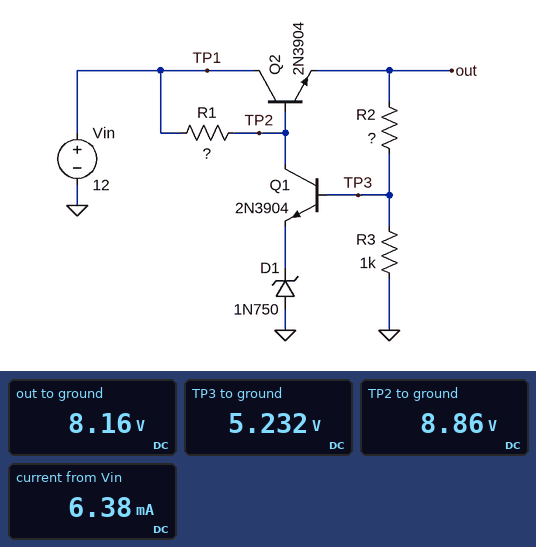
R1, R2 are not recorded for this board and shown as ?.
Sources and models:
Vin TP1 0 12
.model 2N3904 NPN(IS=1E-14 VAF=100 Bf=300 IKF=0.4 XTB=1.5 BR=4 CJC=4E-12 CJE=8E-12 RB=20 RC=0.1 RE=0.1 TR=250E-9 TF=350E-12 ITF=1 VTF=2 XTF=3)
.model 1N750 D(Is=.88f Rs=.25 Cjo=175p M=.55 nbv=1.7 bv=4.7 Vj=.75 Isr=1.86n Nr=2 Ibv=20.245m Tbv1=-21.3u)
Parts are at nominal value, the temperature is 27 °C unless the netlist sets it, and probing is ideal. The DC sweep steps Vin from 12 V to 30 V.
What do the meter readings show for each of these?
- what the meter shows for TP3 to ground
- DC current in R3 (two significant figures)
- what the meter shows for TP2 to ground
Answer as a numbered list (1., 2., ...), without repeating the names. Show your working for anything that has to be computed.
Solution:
1. 5.232 V
2. (5.232 V) / 1 kΩ = 5.2 mA
3. 8.86 V
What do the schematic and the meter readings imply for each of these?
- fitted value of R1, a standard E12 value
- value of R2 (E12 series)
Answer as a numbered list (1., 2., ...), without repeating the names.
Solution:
1. 2.7 kΩ
2. 560 Ω
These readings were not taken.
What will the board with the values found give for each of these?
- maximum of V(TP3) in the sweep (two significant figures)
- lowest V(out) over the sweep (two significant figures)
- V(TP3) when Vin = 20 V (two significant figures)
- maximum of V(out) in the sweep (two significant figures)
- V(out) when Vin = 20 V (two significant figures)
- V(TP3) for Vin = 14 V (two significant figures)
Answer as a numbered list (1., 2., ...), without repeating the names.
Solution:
1. 5.4 V
2. 8.2 V
3. 5.3 V
4. 8.4 V
5. 8.3 V
6. 5.3 V
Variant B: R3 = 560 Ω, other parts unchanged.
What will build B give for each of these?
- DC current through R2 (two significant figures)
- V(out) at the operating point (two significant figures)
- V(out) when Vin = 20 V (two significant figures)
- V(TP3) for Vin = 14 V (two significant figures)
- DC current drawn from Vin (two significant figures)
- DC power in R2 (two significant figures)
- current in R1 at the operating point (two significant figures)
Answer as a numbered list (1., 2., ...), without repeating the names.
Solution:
1. 9.2 mA
2. 10 V
3. 11 V
4. 5.2 V
5. 9.5 mA
6. 47 mW
7. 370 µA
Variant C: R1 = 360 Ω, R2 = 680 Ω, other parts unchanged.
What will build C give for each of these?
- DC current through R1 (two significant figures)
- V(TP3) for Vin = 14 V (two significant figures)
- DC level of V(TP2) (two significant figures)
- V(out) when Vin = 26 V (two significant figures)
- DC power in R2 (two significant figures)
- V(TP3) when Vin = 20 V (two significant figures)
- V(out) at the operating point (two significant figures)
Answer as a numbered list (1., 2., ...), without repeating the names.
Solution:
1. 6.4 mA
2. 5.4 V
3. 9.7 V
4. 9.4 V
5. 20 mW
6. 5.5 V
7. 9.0 V
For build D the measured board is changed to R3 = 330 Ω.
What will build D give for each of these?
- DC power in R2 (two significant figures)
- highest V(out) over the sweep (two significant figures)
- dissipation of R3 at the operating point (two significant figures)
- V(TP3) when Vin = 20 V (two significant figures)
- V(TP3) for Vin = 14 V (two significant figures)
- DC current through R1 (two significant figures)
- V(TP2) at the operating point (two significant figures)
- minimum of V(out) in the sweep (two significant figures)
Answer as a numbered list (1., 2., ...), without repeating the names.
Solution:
1. 88 mW
2. 14 V
3. 52 mW
4. 5.3 V
5. 4.9 V
6. 43 µA
7. 12 V
8. 11 V
